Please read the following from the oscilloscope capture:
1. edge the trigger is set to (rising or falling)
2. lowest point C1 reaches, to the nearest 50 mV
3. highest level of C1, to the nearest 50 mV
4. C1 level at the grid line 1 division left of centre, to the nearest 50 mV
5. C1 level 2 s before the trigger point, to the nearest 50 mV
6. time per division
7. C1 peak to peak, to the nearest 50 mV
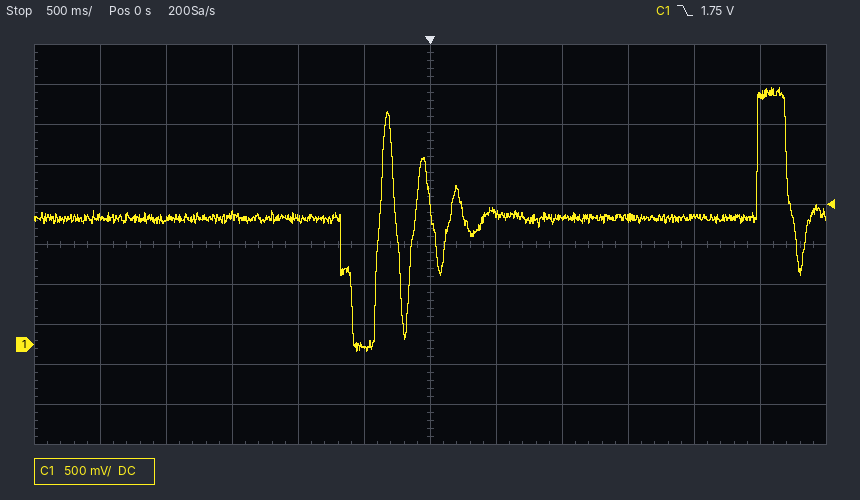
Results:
falling
-100 mV
3.20 V
-50 mV
1.55 V
500 ms
3.30 V
